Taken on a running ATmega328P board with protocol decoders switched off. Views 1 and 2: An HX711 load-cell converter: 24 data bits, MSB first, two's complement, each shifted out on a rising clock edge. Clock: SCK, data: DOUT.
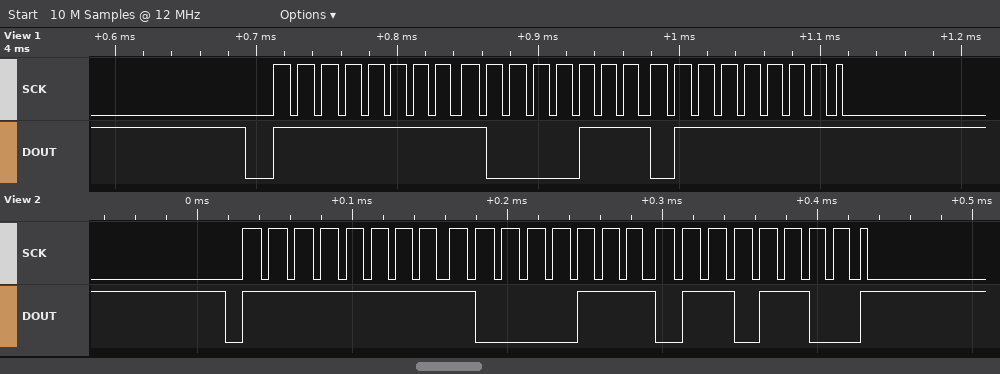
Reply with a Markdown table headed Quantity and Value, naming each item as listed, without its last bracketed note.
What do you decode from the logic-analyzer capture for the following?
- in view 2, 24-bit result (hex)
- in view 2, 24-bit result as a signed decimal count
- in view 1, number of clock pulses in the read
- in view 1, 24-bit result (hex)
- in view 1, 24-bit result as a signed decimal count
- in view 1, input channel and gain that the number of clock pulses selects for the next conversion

| Quantity | Value |
|---|---|
| in view 2, 24-bit result | 0xFF876C |
| in view 2, 24-bit result as a signed decimal count | -30868 |
| in view 1, number of clock pulses in the read | 25 |
| in view 1, 24-bit result | 0xFF877F |
| in view 1, 24-bit result as a signed decimal count | -30849 |
| in view 1, input channel and gain that the number of clock pulses selects for the next conversion | channel A, gain 128 |
